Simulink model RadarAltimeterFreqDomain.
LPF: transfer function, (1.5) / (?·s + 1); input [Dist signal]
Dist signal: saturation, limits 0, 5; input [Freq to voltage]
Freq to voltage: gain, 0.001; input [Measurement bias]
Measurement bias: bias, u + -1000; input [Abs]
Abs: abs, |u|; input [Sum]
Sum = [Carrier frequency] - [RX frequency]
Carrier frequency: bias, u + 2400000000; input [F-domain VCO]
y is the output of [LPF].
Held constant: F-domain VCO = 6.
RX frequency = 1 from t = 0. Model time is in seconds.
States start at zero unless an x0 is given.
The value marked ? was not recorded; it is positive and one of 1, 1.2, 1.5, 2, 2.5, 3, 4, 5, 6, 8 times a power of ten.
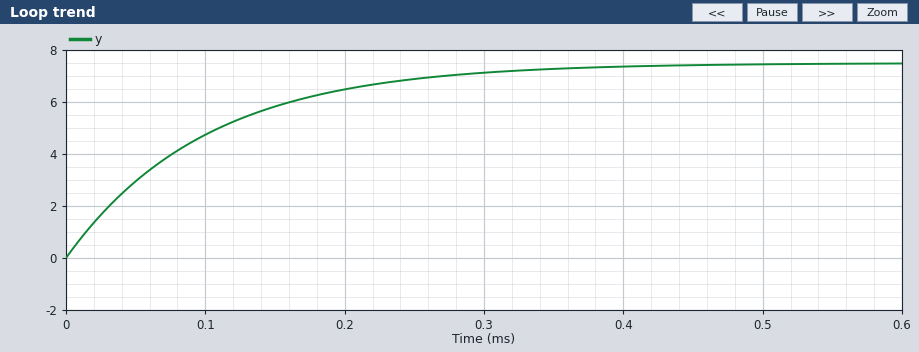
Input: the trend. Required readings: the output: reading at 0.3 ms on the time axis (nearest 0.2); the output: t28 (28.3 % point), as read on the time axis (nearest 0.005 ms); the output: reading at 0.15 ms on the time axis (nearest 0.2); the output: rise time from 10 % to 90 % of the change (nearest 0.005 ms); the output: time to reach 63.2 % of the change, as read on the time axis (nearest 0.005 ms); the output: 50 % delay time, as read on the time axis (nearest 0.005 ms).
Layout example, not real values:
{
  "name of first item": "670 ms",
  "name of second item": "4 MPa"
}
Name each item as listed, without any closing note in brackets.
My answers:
{
  "the output: reading at 0.3 ms on the time axis": "7.2",
  "the output: t28 (28.3 % point), as read on the time axis": "0.035 ms",
  "the output: reading at 0.15 ms on the time axis": "5.8",
  "the output: rise time from 10 % to 90 % of the change": "0.220 ms",
  "the output: time to reach 63.2 % of the change, as read on the time axis": "0.100 ms",
  "the output: 50 % delay time, as read on the time axis": "0.070 ms"
}
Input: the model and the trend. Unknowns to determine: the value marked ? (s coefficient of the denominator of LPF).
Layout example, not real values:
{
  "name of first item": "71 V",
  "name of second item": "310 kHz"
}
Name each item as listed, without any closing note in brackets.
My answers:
{
  "the value marked ?": "0.0001"
}
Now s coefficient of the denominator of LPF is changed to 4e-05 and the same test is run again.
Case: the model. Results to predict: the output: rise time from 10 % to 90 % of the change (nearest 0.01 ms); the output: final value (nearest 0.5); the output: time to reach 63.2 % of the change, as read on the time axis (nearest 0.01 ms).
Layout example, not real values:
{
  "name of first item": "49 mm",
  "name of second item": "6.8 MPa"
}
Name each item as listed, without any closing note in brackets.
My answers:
{
  "the output: rise time from 10 % to 90 % of the change": "0.09 ms",
  "the output: final value": "7.5",
  "the output: time to reach 63.2 % of the change, as read on the time axis": "0.04 ms"
}
